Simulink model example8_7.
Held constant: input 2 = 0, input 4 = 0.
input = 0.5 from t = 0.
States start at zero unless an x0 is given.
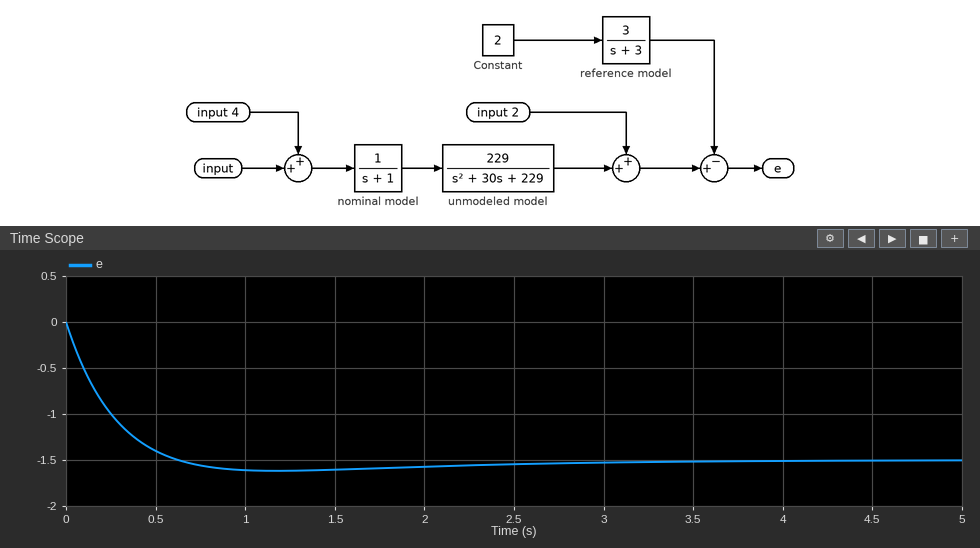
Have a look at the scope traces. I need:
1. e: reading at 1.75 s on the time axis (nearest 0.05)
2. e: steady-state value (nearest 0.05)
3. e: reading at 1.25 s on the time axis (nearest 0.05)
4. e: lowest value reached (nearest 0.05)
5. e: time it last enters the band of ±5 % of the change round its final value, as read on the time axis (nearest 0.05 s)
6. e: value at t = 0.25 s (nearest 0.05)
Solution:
-1.60
-1.50
-1.60
-1.60
1.95 s
-1.00
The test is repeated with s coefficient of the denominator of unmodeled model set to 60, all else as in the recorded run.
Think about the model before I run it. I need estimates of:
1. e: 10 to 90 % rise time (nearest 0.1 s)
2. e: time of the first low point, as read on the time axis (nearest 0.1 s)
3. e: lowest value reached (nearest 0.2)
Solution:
0.4 s
1.1 s
-1.6
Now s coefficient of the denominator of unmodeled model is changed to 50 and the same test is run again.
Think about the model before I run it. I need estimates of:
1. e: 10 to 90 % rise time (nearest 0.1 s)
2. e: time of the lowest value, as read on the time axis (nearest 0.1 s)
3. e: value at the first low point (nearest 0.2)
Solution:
0.4 s
1.1 s
-1.6
